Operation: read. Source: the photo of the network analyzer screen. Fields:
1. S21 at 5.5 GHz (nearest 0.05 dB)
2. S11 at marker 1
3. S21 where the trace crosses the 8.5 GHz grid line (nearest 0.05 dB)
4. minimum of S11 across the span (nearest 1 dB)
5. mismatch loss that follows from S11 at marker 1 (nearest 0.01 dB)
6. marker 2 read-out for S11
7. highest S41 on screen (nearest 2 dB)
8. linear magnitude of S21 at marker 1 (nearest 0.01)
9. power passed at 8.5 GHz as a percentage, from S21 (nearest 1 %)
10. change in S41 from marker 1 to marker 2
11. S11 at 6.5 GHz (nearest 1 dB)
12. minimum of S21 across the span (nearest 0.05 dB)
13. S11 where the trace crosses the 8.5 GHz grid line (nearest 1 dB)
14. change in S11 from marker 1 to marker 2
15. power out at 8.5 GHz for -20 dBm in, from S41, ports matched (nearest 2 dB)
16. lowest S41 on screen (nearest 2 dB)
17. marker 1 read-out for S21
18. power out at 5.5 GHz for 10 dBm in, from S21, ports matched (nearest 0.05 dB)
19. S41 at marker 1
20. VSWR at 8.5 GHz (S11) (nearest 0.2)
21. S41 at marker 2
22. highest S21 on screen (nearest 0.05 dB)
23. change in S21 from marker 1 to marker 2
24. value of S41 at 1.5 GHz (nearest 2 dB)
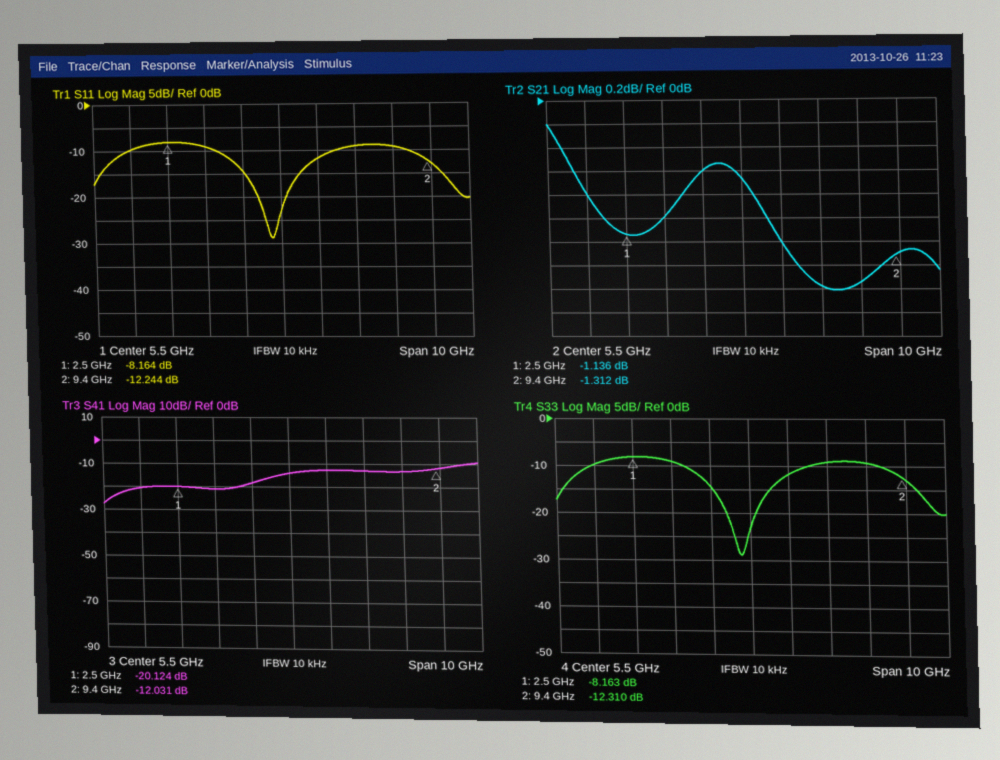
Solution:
-0.65 dB
-8.164 dB
-1.55 dB
-29 dB
0.72 dB
-12.244 dB
-10 dB
0.88
70 %
8.093 dB
-12 dB
-1.60 dB
-9 dB
-4.080 dB
-34 dBm
-28 dB
-1.136 dB
9.35 dBm
-20.124 dB
2.0
-12.031 dB
-0.20 dB
-0.176 dB
-20 dB
